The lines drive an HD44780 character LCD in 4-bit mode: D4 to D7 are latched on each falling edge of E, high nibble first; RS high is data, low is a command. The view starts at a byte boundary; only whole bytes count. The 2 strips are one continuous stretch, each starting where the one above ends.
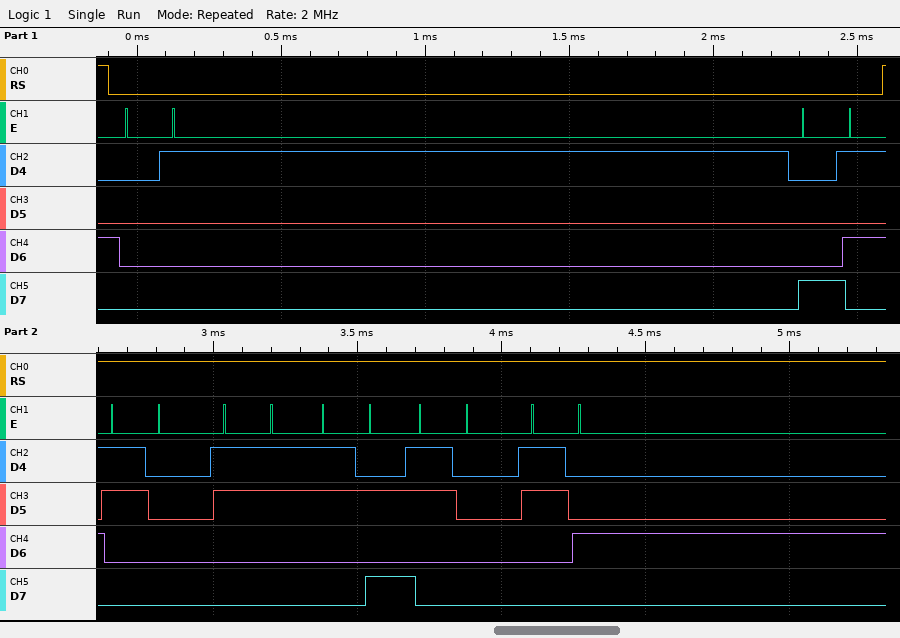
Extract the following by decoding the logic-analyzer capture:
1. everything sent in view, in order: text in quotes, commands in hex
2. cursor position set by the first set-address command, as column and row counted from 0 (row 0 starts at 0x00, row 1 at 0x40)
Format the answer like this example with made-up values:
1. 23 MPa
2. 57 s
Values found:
1. 0x01 0x85 "03:04"
2. column 5, row 0
